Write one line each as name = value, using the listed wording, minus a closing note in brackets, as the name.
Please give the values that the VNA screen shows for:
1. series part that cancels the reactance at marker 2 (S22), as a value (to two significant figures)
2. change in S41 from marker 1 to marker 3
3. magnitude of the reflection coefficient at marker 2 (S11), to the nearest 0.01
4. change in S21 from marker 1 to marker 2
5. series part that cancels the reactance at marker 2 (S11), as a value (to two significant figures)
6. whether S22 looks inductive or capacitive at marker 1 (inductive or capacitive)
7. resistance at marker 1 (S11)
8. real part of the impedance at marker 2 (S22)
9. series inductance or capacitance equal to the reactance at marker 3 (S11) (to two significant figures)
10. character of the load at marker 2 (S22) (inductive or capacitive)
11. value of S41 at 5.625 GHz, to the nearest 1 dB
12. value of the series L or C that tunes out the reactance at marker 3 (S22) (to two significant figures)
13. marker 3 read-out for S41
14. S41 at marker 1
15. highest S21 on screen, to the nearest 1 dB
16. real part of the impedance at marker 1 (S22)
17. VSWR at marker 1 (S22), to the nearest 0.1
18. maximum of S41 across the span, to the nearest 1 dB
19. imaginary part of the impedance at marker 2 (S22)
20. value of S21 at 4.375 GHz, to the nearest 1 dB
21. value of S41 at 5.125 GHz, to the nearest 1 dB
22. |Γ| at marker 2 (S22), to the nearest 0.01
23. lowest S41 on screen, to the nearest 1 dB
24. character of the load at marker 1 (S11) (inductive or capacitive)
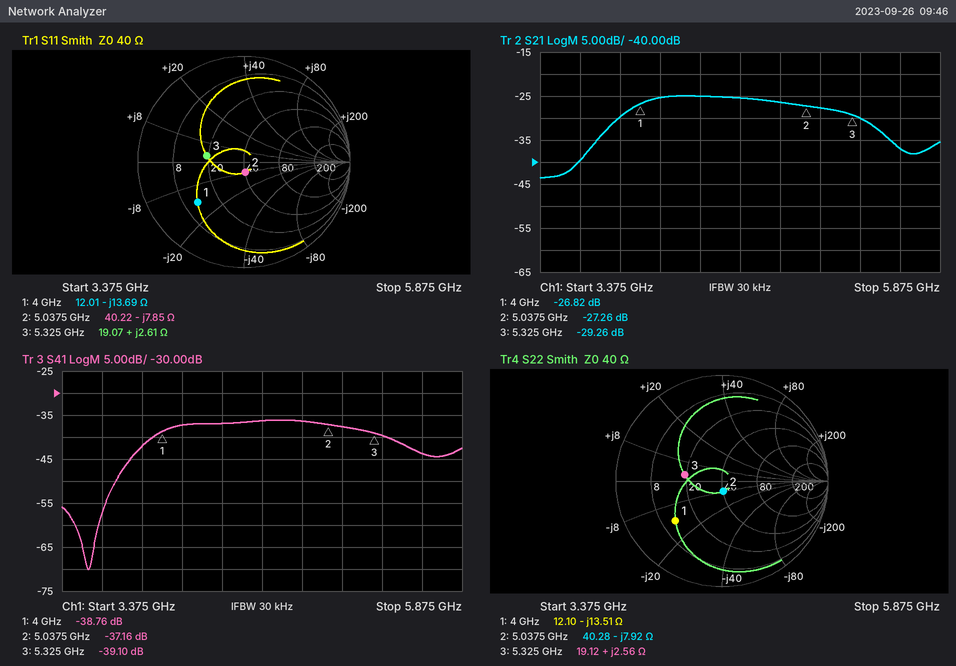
series part that cancels the reactance at marker 2 (S22), as a value = 250 pH
change in S41 from marker 1 to marker 3 = -0.34 dB
magnitude of the reflection coefficient at marker 2 (S11), to the nearest 0.01 = 0.10
change in S21 from marker 1 to marker 2 = -0.44 dB
series part that cancels the reactance at marker 2 (S11), as a value = 250 pH
whether S22 looks inductive or capacitive at marker 1 = capacitive
resistance at marker 1 = 12.01 Ω
real part of the impedance at marker 2 = 40.28 Ω
series inductance or capacitance equal to the reactance at marker 3 (S11) = 78 pH
character of the load at marker 2 (S22) = capacitive
value of S41 at 5.625 GHz, to the nearest 1 dB = -44 dB
value of the series L or C that tunes out the reactance at marker 3 (S22) = 12 pF
marker 3 read-out for S41 = -39.10 dB
S41 at marker 1 = -38.76 dB
highest S21 on screen, to the nearest 1 dB = -25 dB
real part of the impedance at marker 1 = 12.10 Ω
VSWR at marker 1 (S22), to the nearest 0.1 = 3.7
maximum of S41 across the span, to the nearest 1 dB = -36 dB
imaginary part of the impedance at marker 2 = -7.92 Ω
value of S21 at 4.375 GHz, to the nearest 1 dB = -25 dB
value of S41 at 5.125 GHz, to the nearest 1 dB = -38 dB
|Γ| at marker 2 (S22), to the nearest 0.01 = 0.10
lowest S41 on screen, to the nearest 1 dB = -70 dB
character of the load at marker 1 (S11) = capacitive
